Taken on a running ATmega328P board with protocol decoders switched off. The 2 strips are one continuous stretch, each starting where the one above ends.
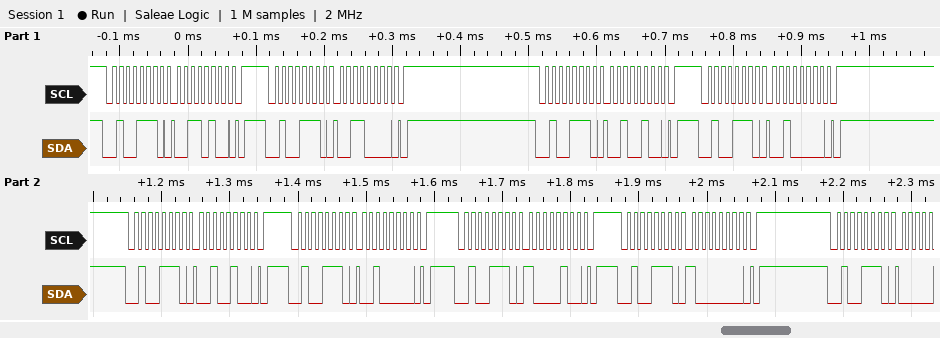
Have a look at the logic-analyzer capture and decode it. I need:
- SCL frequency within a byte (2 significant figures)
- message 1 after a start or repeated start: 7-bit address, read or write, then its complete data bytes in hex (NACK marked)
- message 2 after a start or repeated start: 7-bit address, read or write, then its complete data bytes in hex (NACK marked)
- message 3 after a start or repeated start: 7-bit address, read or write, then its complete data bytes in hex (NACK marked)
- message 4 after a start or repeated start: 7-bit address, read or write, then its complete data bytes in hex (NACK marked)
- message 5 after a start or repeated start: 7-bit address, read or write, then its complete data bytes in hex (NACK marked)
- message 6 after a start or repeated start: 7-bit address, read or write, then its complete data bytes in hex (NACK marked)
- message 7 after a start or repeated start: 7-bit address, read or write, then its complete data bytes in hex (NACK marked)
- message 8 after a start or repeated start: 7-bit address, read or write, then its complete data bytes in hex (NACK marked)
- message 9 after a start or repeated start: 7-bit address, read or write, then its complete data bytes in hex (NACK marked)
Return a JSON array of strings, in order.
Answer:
["100 kHz", "0x27 write: 34", "0x27 write: 30", "0x27 write: 24", "0x27 write: 20", "0x27 write: 24", "0x27 write: 20", "0x27 write: 84", "0x27 write: 80", "0x27 write"]
